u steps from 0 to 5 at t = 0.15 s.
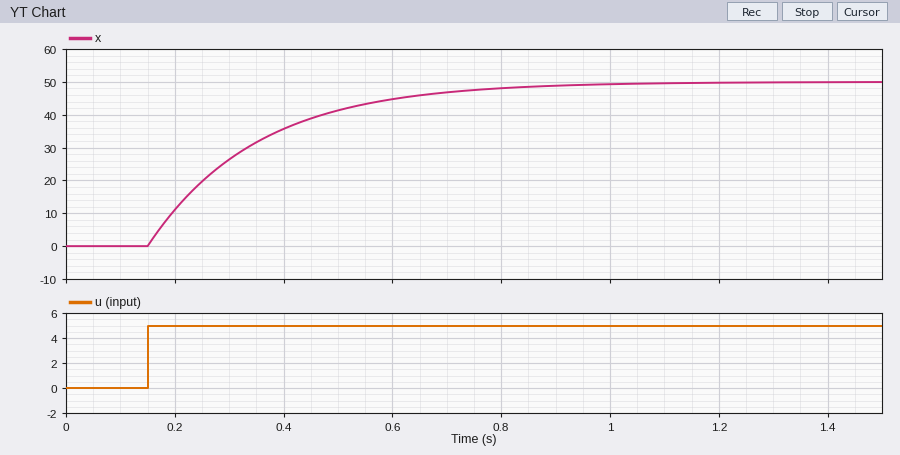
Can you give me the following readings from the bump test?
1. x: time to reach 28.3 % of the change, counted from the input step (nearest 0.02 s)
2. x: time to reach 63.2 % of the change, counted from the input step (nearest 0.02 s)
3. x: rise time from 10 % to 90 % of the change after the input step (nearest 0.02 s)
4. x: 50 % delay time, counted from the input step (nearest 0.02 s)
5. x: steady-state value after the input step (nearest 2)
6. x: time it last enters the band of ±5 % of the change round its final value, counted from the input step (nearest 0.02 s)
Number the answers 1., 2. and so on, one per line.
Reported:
1. 0.06 s
2. 0.20 s
3. 0.44 s
4. 0.14 s
5. 50
6. 0.60 s
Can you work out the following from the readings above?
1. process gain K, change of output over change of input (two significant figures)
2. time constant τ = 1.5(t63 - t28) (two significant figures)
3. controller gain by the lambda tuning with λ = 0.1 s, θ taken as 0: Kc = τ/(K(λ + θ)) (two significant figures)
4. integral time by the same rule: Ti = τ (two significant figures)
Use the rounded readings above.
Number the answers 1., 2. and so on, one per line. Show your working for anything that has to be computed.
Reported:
1. (50 - 0) / 5 = 10
2. 1.5 × (0.2 - 0.06) = 0.21 s
3. 0.21 / (10 × (0.1 + 0)) = 0.21
4. 0.21 s
